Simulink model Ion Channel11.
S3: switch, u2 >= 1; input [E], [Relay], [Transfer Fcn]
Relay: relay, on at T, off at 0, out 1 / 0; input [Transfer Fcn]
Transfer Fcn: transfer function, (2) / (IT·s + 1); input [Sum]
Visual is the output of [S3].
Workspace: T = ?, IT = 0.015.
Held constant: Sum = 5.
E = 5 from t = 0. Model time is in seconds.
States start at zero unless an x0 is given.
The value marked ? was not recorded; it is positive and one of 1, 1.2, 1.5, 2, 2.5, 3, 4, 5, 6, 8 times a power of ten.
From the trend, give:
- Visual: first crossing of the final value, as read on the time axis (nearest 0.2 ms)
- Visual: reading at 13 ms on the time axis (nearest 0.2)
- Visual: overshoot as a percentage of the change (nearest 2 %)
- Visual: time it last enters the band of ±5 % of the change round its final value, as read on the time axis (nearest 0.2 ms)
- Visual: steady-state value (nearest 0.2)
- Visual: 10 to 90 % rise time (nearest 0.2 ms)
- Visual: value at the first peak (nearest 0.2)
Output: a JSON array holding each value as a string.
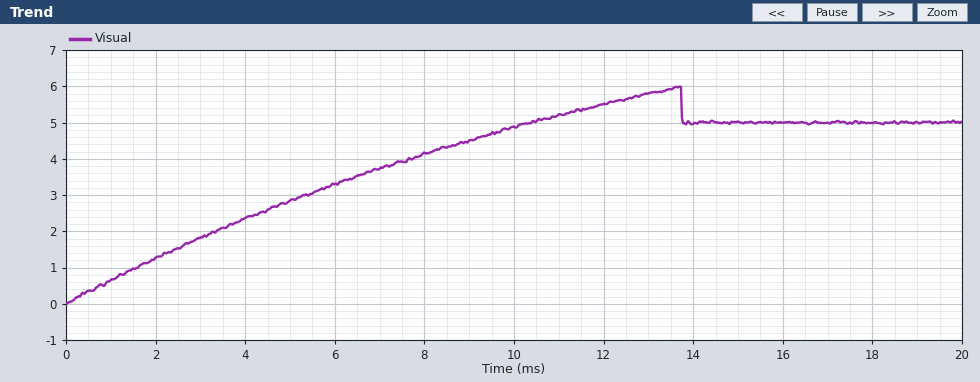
["10.4 ms", "5.8", "20 %", "13.8 ms", "5.0", "8.2 ms", "6.0"]
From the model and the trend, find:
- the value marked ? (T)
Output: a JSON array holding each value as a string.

["6"]
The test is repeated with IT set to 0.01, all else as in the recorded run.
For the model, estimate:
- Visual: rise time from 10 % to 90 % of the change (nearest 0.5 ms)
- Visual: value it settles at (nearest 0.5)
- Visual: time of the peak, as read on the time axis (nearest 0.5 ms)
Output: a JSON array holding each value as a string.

["5.5 ms", "5.0", "9.0 ms"]
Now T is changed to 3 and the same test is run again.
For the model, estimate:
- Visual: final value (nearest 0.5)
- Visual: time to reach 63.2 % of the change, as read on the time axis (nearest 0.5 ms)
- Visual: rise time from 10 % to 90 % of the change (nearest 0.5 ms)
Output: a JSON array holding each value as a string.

["5.0", "5.5 ms", "4.5 ms"]
